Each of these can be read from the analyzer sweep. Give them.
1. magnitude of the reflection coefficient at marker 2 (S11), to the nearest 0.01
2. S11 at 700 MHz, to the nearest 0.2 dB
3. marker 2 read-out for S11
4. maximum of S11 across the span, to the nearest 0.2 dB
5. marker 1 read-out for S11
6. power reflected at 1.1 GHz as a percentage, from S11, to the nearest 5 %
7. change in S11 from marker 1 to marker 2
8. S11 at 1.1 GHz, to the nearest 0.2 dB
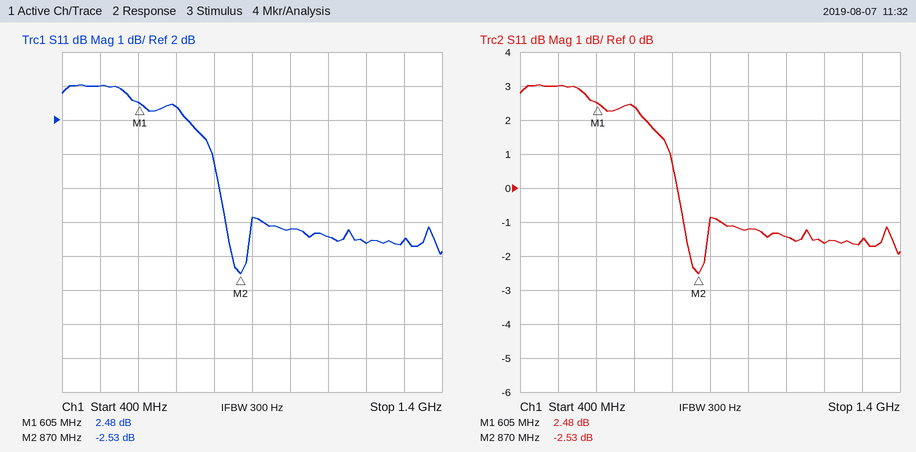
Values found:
0.75
2.4 dB
-2.53 dB
3.0 dB
2.48 dB
70 %
-5.01 dB
-1.4 dB
